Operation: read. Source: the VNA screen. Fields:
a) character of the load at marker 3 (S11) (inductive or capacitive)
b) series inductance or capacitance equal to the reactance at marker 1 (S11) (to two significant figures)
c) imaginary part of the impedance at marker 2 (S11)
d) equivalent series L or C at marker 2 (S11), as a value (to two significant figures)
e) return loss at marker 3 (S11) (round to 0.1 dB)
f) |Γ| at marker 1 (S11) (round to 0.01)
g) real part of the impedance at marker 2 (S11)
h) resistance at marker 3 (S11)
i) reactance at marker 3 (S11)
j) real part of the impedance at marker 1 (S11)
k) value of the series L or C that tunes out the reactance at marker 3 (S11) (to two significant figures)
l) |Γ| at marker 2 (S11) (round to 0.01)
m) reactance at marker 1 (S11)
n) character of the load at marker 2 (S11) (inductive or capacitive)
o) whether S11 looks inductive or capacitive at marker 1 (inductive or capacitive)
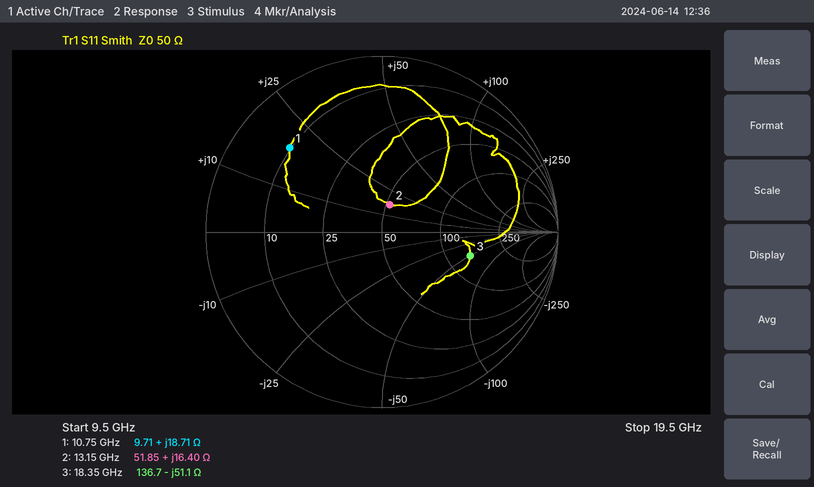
capacitive
280 pH
+16.40 Ω
200 pH
5.7 dB
0.71
51.85 Ω
136.7 Ω
-51.1 Ω
9.71 Ω
440 pH
0.16
+18.71 Ω
inductive
inductive
